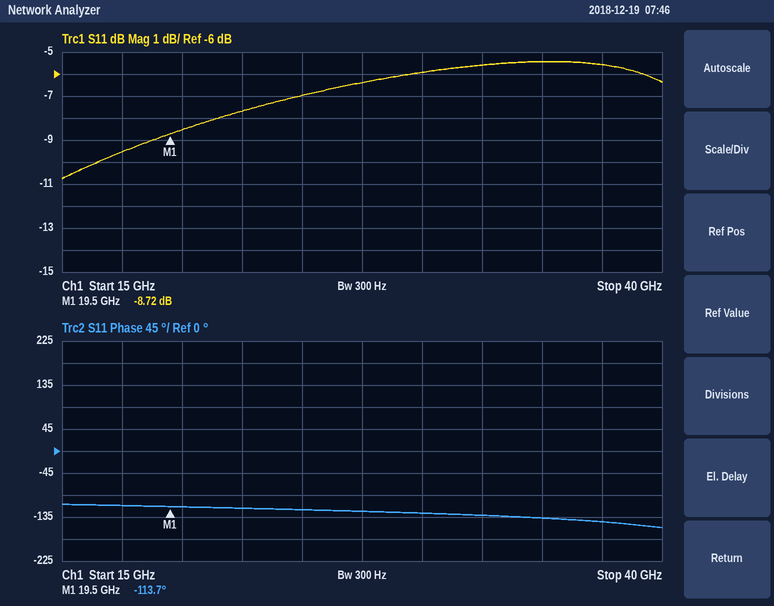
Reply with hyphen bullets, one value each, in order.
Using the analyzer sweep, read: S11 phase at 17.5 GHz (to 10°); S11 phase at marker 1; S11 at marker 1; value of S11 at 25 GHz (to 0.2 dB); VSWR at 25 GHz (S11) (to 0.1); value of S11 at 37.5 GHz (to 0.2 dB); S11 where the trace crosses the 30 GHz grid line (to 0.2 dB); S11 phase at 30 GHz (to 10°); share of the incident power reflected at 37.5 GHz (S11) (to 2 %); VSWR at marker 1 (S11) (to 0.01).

- -110°
- -113.7°
- -8.72 dB
- -7.0 dB
- 2.6
- -5.6 dB
- -6.0 dB
- -130°
- 28 %
- 2.16
